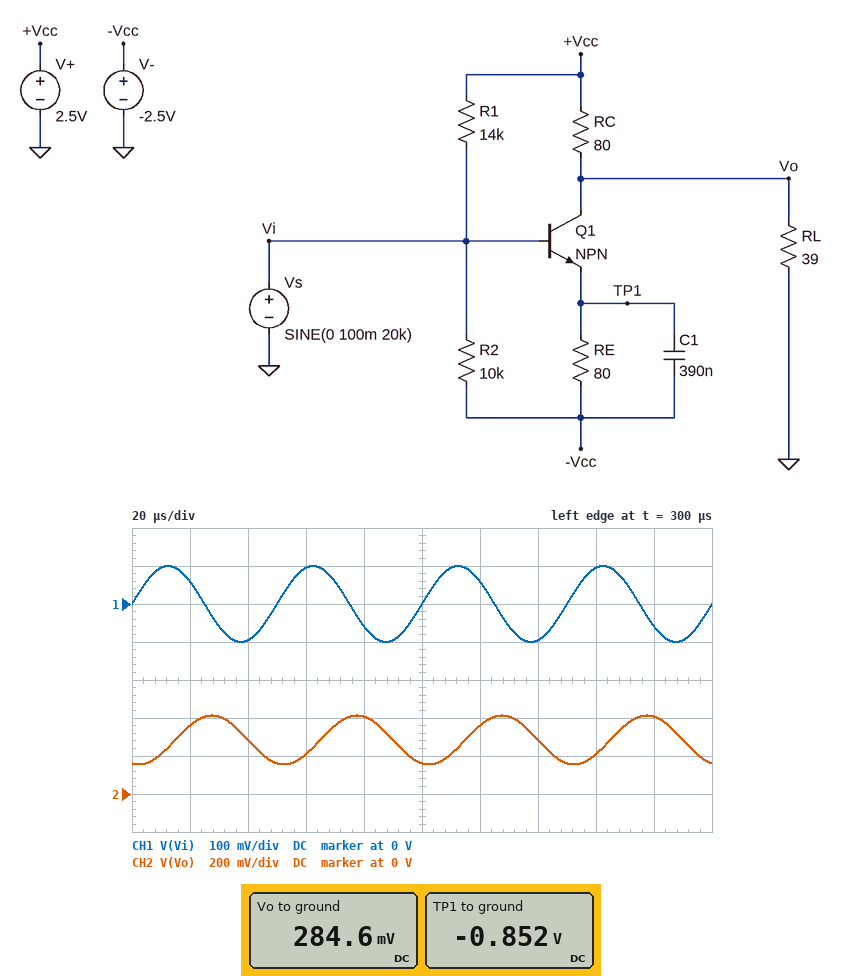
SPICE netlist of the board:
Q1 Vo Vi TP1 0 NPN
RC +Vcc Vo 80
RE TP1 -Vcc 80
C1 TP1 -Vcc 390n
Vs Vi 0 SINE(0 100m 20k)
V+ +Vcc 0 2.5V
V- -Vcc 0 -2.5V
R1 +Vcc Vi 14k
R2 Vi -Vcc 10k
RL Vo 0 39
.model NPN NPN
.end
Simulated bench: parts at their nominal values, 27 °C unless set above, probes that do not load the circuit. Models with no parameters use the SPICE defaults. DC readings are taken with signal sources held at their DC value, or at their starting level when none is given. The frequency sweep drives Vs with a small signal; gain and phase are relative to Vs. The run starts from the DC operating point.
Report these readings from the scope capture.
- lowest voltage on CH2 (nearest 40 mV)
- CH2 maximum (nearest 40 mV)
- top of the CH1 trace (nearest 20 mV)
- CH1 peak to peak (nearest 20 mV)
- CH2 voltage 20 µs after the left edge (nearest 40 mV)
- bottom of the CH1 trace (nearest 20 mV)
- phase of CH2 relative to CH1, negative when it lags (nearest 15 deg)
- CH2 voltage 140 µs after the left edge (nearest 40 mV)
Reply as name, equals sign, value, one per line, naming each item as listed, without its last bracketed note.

lowest voltage on CH2 = 160 mV
CH2 maximum = 400 mV
top of the CH1 trace = 100 mV
CH1 peak to peak = 200 mV
CH2 voltage 20 µs after the left edge = 360 mV
bottom of the CH1 trace = -100 mV
phase of CH2 relative to CH1, negative when it lags = -105 deg
CH2 voltage 140 µs after the left edge = 280 mV
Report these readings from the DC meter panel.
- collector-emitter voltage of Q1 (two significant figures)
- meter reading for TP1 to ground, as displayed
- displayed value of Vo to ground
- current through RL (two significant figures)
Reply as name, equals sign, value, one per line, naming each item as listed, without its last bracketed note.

collector-emitter voltage of Q1 = 1.1 V
meter reading for TP1 to ground, as displayed = -0.852 V
displayed value of Vo to ground = 284.6 mV
current through RL = 7.3 mA
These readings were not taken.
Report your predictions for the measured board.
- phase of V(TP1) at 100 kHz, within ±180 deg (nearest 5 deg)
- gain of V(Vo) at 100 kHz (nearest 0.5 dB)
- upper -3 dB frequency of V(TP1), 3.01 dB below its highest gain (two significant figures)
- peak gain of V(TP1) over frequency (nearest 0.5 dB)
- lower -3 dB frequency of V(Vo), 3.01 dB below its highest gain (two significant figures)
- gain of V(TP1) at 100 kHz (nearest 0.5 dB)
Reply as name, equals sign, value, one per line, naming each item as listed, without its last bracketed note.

phase of V(TP1) at 100 kHz, within ±180 deg = -15 deg
gain of V(Vo) at 100 kHz = 15.5 dB
upper -3 dB frequency of V(TP1), 3.01 dB below its highest gain = 330 kHz
peak gain of V(TP1) over frequency = 0 dB
lower -3 dB frequency of V(Vo), 3.01 dB below its highest gain = 330 kHz
gain of V(TP1) at 100 kHz = -0.5 dB
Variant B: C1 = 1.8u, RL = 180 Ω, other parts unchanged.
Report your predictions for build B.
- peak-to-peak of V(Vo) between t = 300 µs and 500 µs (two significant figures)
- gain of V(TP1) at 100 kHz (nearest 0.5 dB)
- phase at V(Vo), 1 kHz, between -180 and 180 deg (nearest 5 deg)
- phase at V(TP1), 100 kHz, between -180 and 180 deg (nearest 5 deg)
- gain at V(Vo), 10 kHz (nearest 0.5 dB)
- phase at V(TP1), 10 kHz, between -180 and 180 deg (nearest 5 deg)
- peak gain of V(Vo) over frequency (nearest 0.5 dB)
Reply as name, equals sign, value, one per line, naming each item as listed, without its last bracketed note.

peak-to-peak of V(Vo) between t = 300 µs and 500 µs = 2.2 V
gain of V(TP1) at 100 kHz = -5.0 dB
phase at V(Vo), 1 kHz, between -180 and 180 deg = -140 deg
phase at V(TP1), 100 kHz, between -180 and 180 deg = -55 deg
gain at V(Vo), 10 kHz = 15.5 dB
phase at V(TP1), 10 kHz, between -180 and 180 deg = -10 deg
peak gain of V(Vo) over frequency = 33.0 dB
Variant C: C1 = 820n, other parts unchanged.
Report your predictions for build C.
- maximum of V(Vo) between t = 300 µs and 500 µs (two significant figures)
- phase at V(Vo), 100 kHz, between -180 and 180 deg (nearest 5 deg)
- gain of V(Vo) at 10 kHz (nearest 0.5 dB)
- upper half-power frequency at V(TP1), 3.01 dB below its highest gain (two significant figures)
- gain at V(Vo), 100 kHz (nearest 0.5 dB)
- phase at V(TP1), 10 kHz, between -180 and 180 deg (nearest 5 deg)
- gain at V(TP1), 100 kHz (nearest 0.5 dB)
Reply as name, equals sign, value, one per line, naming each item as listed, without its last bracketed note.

maximum of V(Vo) between t = 300 µs and 500 µs = 540 mV
phase at V(Vo), 100 kHz, between -180 and 180 deg = -125 deg
gain of V(Vo) at 10 kHz = 2.5 dB
upper half-power frequency at V(TP1), 3.01 dB below its highest gain = 160 kHz
gain at V(Vo), 100 kHz = 21.0 dB
phase at V(TP1), 10 kHz, between -180 and 180 deg = -5 deg
gain at V(TP1), 100 kHz = -1.5 dB
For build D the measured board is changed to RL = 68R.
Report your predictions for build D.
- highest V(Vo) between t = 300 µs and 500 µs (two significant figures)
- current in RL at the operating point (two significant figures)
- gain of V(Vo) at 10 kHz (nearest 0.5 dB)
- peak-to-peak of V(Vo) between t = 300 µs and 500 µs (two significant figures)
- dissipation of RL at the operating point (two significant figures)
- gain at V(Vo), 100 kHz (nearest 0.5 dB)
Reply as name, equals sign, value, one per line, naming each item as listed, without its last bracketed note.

highest V(Vo) between t = 300 µs and 500 µs = 580 mV
current in RL at the operating point = 5.9 mA
gain of V(Vo) at 10 kHz = 0 dB
peak-to-peak of V(Vo) between t = 300 µs and 500 µs = 360 mV
dissipation of RL at the operating point = 2.3 mW
gain at V(Vo), 100 kHz = 18.5 dB
